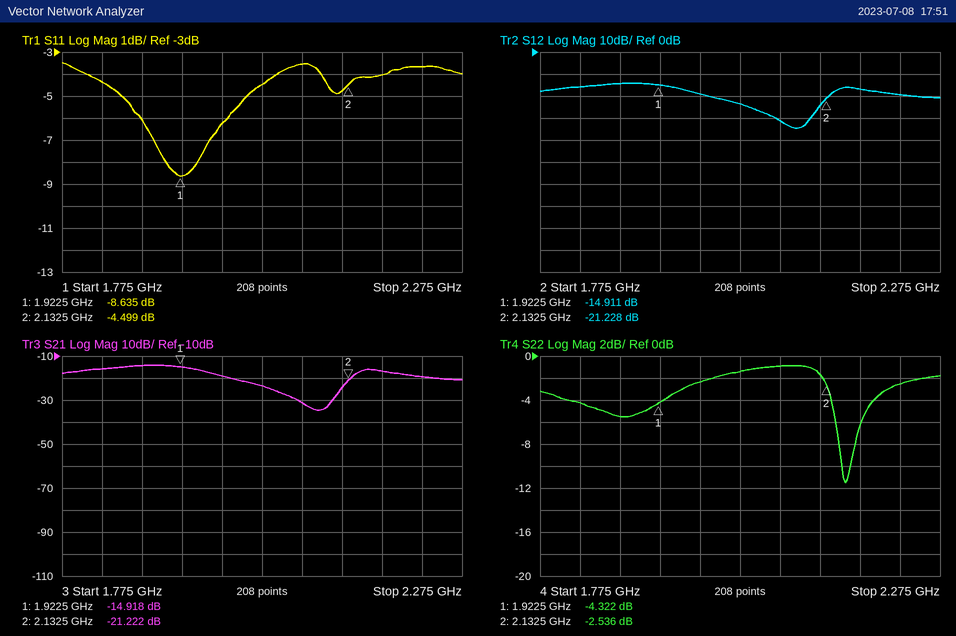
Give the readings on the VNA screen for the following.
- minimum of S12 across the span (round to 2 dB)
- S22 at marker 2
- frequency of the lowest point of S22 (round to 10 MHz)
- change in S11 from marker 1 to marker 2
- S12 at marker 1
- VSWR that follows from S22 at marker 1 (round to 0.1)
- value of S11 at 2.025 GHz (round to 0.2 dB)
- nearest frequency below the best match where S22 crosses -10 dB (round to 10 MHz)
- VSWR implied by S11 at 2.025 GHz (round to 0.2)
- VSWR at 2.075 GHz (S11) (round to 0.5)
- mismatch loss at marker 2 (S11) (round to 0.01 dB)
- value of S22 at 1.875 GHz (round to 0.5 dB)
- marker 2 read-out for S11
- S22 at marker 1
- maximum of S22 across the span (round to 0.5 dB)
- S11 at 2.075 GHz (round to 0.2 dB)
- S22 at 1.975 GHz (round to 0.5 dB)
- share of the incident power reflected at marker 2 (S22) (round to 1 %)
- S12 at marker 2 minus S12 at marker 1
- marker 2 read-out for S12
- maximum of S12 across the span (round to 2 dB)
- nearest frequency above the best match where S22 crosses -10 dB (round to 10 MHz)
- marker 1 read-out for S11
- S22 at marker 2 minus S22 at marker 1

-34 dB
-2.536 dB
2.16 GHz
4.136 dB
-14.911 dB
4.1
-4.4 dB
2.15 GHz
4.0
5.0
1.90 dB
-5.5 dB
-4.499 dB
-4.322 dB
-1.0 dB
-3.6 dB
-2.5 dB
56 %
-6.317 dB
-21.228 dB
-14 dB
2.16 GHz
-8.635 dB
1.786 dB
